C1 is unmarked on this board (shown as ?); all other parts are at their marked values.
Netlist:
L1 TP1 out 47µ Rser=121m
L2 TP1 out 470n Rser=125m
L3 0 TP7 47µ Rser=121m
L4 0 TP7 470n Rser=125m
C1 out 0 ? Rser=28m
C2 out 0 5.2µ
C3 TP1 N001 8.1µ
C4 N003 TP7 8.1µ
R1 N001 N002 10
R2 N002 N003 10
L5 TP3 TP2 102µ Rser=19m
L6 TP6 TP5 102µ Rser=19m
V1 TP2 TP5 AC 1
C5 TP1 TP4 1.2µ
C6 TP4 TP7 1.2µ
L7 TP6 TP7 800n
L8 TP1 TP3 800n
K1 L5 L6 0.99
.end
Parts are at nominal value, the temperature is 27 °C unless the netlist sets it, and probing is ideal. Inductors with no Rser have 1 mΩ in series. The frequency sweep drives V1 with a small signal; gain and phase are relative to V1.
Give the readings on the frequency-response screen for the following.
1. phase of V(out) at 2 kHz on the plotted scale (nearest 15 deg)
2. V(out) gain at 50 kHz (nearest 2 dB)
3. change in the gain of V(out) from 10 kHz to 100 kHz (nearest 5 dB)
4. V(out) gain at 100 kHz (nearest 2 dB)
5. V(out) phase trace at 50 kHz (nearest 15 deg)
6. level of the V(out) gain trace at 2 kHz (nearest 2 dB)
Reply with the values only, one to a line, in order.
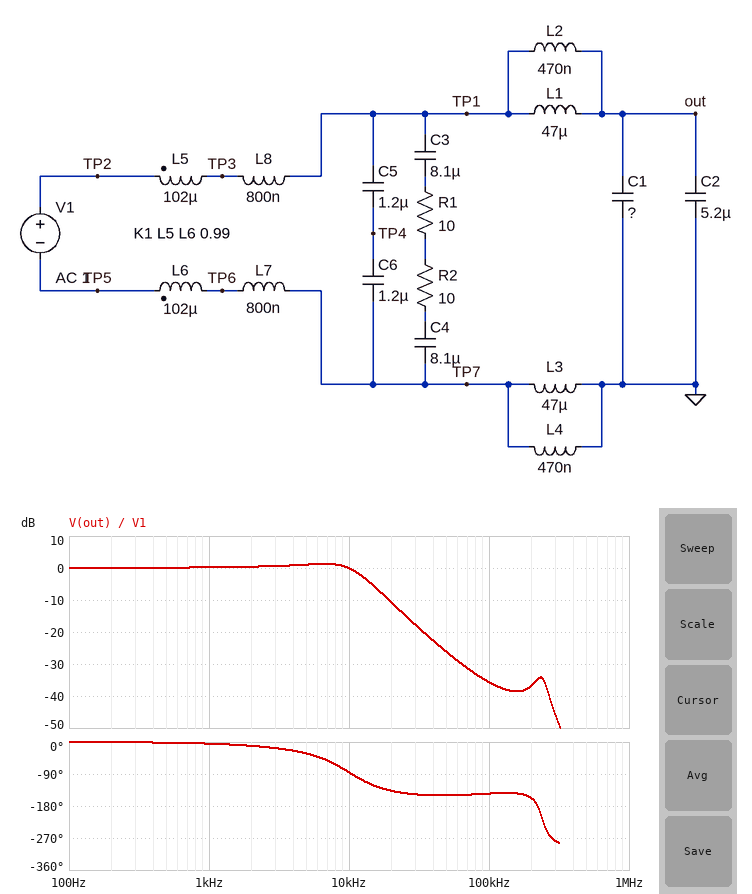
-15 deg
-26 dB
-35 dB
-36 dB
-150 deg
0 dB
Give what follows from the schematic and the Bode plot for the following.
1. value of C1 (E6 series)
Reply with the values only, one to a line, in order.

47 µF
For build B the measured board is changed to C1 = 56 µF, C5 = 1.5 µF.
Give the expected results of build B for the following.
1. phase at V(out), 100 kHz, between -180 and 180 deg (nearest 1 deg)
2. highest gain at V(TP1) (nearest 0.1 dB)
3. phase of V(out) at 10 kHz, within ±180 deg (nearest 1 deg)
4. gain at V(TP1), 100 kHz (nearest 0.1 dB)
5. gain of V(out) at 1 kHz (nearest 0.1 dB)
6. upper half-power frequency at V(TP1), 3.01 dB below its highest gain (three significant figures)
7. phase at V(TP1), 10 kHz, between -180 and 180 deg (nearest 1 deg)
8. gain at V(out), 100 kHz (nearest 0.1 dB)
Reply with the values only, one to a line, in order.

-141 deg
0.9 dB
-93 deg
-17.8 dB
0.3 dB
10.9 kHz
-65 deg
-36.2 dB
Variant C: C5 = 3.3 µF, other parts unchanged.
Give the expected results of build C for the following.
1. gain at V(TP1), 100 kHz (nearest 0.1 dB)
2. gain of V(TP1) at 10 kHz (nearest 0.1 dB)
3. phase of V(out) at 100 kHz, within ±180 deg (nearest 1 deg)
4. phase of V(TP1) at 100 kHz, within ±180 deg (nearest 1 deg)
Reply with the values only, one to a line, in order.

-17.3 dB
0 dB
-148 deg
-32 deg
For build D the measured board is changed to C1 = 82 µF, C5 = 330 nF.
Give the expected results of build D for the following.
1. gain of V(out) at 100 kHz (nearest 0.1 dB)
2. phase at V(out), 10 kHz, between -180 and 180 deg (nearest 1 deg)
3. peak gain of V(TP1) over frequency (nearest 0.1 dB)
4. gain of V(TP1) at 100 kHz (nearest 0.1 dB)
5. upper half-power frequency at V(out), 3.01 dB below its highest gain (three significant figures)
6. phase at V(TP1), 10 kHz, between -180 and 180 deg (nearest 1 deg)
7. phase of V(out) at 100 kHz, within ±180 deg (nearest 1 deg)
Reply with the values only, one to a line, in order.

-38.5 dB
-103 deg
0.4 dB
-18.7 dB
7.92 kHz
-66 deg
-127 deg
